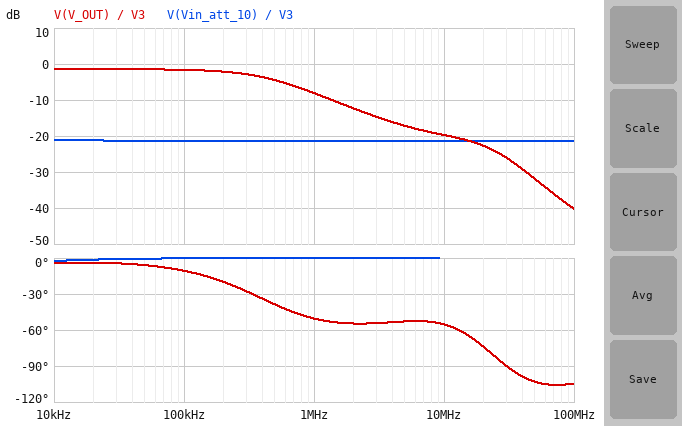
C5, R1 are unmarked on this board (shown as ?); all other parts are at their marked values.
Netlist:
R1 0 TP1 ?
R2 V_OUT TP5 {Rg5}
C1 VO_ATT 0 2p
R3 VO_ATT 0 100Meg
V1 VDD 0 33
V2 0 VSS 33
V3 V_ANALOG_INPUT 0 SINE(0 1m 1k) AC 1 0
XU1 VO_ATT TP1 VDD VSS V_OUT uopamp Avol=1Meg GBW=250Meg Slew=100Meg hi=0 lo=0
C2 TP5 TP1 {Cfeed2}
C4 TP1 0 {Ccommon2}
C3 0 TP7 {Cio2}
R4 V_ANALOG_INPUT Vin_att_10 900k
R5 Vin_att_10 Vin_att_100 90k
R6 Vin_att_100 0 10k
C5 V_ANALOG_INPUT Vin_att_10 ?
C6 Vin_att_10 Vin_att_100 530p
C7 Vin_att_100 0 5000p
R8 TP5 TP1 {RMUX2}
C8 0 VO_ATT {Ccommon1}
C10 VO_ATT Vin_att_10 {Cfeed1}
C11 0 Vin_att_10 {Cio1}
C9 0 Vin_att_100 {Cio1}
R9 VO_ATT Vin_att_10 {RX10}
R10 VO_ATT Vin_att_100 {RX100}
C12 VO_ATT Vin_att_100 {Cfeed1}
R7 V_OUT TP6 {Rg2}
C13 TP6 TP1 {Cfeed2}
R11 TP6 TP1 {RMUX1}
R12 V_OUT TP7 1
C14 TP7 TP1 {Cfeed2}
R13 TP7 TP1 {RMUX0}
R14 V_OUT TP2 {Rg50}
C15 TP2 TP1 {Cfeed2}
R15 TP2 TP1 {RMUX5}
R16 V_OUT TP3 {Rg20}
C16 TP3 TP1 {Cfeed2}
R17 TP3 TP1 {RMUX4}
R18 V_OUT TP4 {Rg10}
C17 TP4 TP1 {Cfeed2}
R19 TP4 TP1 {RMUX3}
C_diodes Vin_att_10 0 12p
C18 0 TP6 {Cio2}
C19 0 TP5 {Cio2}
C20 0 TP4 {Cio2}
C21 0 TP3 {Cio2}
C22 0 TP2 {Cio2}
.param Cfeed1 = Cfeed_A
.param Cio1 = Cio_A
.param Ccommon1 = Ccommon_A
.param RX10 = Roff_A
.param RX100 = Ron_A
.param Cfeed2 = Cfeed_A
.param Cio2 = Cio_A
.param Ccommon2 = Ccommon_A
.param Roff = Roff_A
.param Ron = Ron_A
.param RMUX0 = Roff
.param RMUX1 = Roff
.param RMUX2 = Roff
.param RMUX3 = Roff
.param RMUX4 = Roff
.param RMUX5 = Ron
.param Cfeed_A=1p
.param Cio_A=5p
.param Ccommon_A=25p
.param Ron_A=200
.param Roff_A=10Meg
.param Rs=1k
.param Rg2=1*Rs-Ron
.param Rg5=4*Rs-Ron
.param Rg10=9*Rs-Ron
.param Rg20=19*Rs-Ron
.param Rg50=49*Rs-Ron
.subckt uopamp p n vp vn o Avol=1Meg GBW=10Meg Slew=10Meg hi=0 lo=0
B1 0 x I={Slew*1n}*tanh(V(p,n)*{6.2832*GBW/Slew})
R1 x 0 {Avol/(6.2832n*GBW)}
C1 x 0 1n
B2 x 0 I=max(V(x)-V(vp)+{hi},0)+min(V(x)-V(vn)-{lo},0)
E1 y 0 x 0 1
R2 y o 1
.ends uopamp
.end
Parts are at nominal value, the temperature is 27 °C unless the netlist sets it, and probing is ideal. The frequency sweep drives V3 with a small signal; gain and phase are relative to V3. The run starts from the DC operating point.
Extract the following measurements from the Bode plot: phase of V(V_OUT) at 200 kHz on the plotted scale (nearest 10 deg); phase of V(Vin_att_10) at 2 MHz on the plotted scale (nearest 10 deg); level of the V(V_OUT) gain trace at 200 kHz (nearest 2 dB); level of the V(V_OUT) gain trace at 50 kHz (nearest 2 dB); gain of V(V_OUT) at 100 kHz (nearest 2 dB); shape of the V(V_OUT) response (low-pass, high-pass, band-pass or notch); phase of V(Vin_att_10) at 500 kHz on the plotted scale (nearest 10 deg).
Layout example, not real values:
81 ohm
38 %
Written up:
-20 deg
0 deg
-2 dB
-2 dB
-2 dB
low-pass
0 deg
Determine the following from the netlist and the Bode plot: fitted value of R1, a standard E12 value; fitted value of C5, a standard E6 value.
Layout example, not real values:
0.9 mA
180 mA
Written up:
470 Ω
47 pF
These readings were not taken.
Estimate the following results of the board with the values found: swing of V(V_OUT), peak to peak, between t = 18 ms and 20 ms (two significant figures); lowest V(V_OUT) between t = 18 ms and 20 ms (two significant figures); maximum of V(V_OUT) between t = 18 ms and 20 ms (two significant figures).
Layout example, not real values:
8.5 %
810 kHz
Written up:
2.0 mV
-1.0 mV
1.0 mV
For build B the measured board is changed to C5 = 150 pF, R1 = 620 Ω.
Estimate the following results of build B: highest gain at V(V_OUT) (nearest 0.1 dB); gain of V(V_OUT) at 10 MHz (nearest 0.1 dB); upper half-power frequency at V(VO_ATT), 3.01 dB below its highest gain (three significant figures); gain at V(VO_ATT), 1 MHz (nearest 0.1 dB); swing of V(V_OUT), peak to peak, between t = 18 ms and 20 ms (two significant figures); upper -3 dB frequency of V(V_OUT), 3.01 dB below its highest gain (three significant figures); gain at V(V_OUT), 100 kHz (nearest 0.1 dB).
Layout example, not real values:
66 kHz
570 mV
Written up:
4.7 dB
-11.4 dB
33.3 MHz
-33.1 dB
1.9 mV
528 kHz
4.6 dB
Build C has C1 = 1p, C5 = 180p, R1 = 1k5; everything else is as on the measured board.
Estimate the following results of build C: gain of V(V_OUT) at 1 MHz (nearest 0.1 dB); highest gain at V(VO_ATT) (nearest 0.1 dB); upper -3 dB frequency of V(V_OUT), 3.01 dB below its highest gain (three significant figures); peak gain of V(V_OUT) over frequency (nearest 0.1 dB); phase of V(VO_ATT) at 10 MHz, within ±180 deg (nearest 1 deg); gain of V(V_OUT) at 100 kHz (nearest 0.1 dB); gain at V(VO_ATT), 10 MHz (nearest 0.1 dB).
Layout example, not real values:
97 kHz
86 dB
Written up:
-6.9 dB
-31.9 dB
600 kHz
-1.6 dB
-11 deg
-1.7 dB
-32.3 dB
